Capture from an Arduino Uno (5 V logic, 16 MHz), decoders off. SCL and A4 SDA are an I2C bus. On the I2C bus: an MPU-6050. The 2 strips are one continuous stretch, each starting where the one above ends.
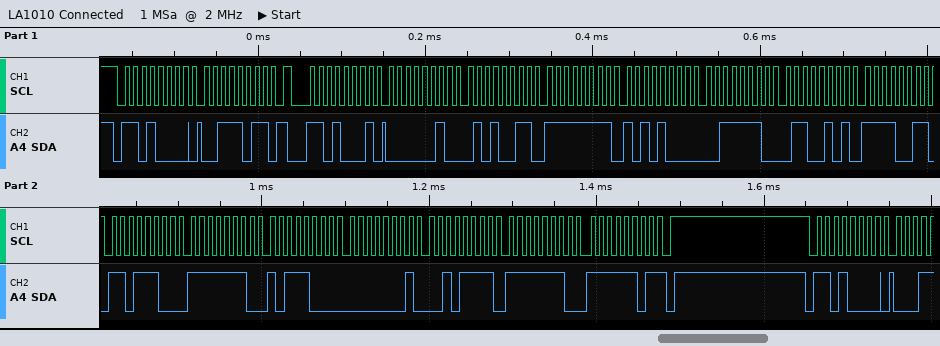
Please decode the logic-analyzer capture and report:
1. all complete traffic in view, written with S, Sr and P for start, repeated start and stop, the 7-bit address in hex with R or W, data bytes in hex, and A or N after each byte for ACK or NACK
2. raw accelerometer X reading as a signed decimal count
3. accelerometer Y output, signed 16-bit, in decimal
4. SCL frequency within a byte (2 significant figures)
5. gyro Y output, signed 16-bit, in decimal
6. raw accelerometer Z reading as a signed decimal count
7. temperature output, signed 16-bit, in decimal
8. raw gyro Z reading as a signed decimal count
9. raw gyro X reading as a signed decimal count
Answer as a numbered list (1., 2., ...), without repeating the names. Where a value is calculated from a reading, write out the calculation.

1. S 68W A 3B A Sr 68R A 02 A 53 A FF A A8 A 3E A 65 A F3 A DC A FE A B8 A 01 A 2F A FE A FD N P S 68W A
2. 0x0253 = 595
3. 0xFFA8 = -88
4. 100 kHz
5. 0x012F = 303
6. 0x3E65 = 15973
7. 0xF3DC = -3108
8. 0xFEFD = -259
9. 0xFEB8 = -328
